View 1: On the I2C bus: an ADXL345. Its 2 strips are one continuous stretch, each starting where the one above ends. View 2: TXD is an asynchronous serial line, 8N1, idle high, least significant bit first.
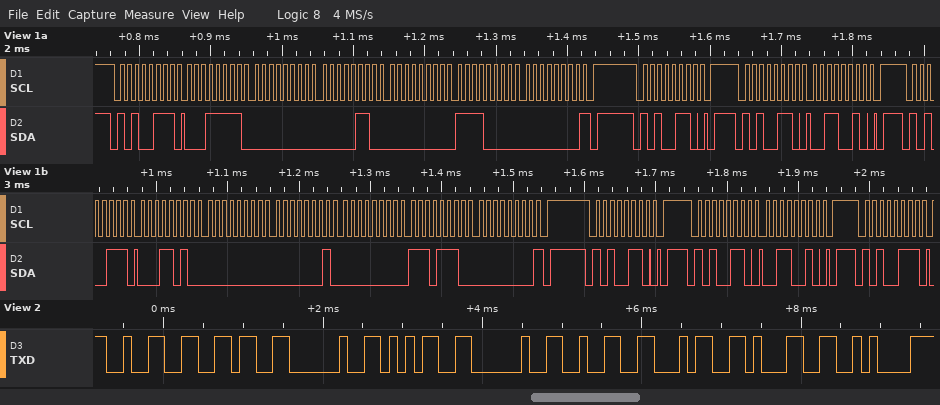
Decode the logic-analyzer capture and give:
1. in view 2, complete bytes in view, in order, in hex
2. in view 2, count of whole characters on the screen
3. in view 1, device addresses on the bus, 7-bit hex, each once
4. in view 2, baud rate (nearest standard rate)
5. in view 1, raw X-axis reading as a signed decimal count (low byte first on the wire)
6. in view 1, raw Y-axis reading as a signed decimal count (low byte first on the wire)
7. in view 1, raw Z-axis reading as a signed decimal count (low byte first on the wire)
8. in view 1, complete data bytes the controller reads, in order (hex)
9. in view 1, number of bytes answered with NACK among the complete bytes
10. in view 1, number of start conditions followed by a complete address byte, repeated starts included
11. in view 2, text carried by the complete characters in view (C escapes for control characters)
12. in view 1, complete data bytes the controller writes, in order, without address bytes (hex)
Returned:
0x32 0x36 0x20 0x35 0x20 0x32 0x34 0x31 0x0A
9
0x53
9600 baud
26
1
238
1F 00 06 00 F0 00 1A 00 01 00 EE 00
2
7
"26 5 241\n"
32 32
